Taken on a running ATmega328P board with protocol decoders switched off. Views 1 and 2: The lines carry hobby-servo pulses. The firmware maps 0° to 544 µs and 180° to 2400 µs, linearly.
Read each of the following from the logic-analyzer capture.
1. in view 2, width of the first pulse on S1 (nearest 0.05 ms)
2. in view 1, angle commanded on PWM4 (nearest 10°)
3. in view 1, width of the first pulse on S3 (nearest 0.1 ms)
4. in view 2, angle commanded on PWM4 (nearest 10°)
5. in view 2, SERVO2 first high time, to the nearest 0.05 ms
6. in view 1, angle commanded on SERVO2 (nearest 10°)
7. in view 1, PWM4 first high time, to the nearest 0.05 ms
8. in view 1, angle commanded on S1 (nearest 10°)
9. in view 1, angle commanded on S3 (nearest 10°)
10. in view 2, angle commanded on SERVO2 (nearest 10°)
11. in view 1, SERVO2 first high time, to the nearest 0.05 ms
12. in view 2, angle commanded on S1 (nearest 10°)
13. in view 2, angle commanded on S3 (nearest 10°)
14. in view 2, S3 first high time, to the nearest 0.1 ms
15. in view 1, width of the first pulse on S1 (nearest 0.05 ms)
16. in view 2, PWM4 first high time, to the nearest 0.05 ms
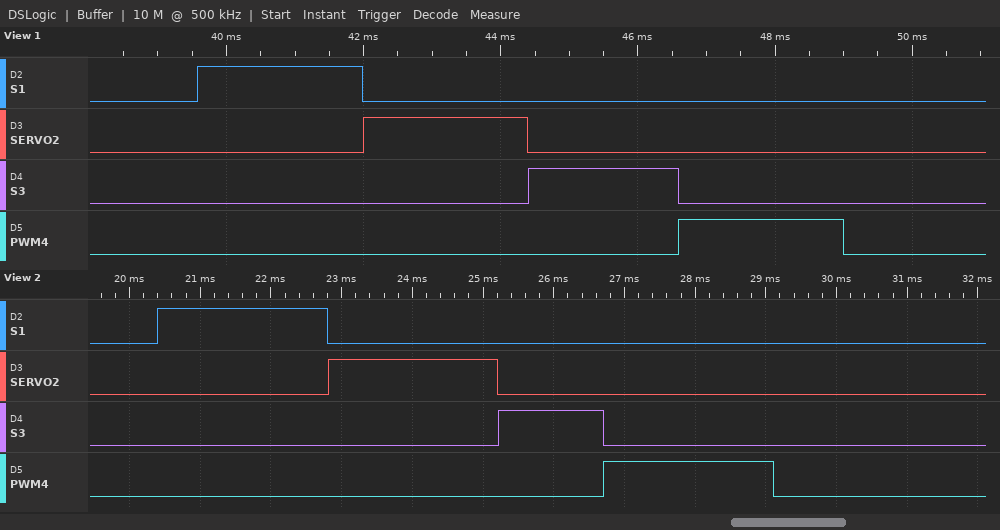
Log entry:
2.40 ms
180°
2.2 ms
180°
2.40 ms
180°
2.40 ms
180°
160°
180°
2.40 ms
180°
90°
1.5 ms
2.40 ms
2.40 ms
